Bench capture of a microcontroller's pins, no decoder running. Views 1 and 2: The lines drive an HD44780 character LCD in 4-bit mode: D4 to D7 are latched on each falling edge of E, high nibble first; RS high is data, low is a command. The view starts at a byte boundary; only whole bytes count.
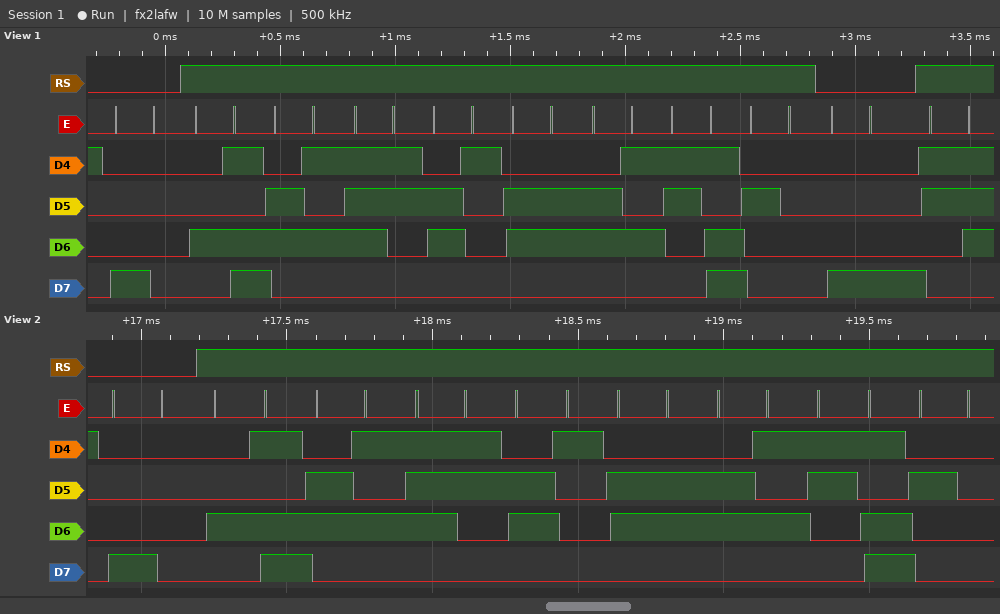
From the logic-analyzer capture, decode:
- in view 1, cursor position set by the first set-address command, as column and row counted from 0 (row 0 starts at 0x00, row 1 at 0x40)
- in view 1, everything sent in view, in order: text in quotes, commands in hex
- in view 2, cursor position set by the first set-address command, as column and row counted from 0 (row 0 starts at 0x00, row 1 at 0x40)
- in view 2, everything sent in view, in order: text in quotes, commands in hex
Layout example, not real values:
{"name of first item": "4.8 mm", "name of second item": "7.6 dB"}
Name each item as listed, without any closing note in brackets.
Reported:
{"in view 1, cursor position set by the first set-address command, as column and row counted from 0": "column 0, row 0", "in view 1, everything sent in view, in order: text in quotes, commands in hex": "0x80 \"Mesafe= \" 0x88 \"7\"", "in view 2, cursor position set by the first set-address command, as column and row counted from 0": "column 0, row 0", "in view 2, everything sent in view, in order: text in quotes, commands in hex": "0x80 \"Mesafe= \""}
